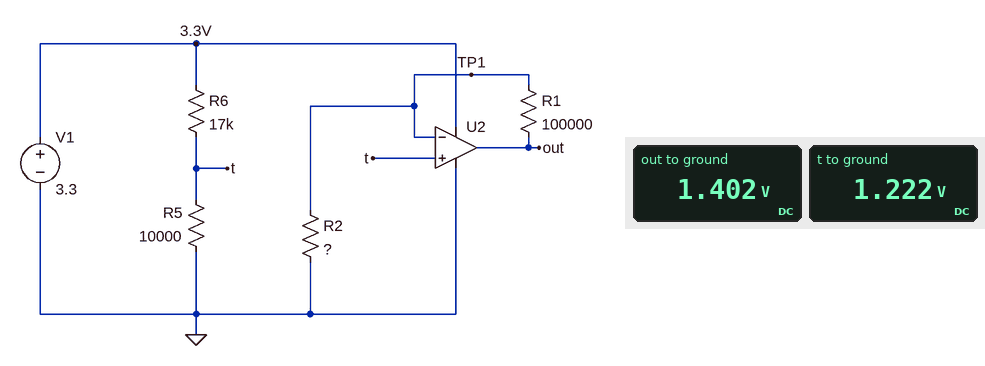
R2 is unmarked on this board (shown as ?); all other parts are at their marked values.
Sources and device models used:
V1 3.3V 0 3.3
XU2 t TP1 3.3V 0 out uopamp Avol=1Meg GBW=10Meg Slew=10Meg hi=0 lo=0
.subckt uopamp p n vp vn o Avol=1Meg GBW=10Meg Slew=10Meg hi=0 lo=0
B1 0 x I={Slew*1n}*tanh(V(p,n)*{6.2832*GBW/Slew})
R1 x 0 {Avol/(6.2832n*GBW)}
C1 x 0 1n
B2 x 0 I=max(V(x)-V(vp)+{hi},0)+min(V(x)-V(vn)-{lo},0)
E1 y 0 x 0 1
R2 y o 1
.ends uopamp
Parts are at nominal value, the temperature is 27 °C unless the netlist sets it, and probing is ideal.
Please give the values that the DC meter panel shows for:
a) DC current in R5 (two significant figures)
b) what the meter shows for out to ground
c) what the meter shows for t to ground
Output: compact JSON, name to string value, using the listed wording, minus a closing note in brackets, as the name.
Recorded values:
{"DC current in R5": "120 µA", "what the meter shows for out to ground": "1.402 V", "what the meter shows for t to ground": "1.222 V"}
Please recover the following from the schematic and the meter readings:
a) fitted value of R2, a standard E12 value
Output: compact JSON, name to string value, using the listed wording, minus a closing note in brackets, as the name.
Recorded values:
{"fitted value of R2, a standard E12 value": "680 kΩ"}
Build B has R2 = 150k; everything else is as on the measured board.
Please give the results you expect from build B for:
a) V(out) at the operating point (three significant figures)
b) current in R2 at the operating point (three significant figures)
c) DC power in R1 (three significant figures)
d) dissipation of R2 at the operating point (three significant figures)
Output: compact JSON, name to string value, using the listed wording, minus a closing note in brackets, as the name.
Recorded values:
{"V(out) at the operating point": "2.04 V", "current in R2 at the operating point": "8.15 µA", "DC power in R1": "6.64 µW", "dissipation of R2 at the operating point": "9.96 µW"}
